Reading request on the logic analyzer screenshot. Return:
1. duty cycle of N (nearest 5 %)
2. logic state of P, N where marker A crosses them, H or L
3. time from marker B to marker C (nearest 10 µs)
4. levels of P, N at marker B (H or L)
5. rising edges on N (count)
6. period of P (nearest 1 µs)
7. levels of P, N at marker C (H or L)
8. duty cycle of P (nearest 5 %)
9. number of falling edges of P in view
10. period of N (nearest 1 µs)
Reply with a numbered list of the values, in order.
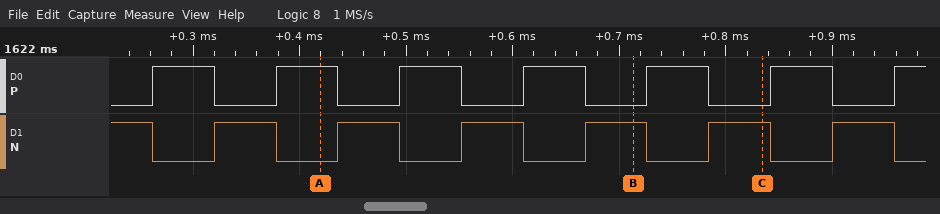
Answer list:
1. 50 %
2. P=H, N=L
3. 120 µs
4. P=L, N=H
5. 6
6. 116 µs
7. P=L, N=H
8. 50 %
9. 6
10. 116 µs
